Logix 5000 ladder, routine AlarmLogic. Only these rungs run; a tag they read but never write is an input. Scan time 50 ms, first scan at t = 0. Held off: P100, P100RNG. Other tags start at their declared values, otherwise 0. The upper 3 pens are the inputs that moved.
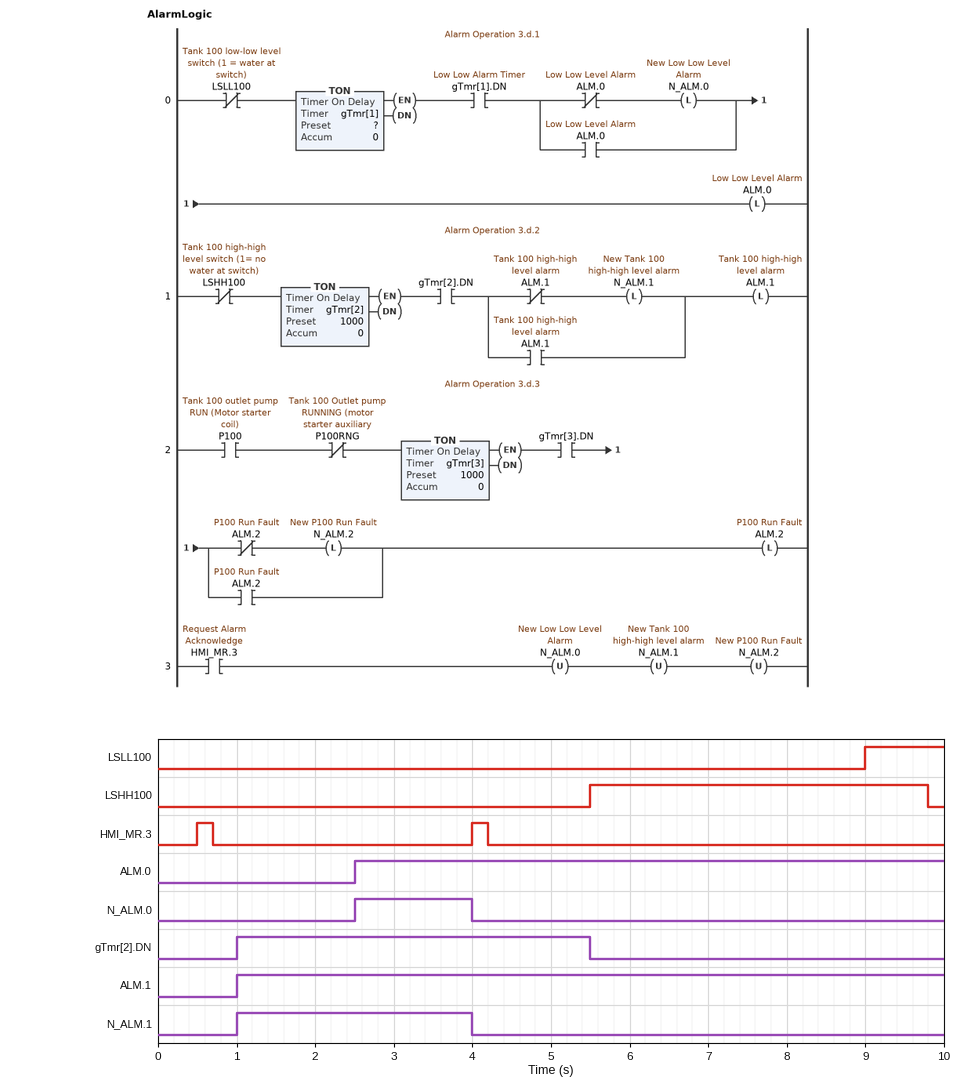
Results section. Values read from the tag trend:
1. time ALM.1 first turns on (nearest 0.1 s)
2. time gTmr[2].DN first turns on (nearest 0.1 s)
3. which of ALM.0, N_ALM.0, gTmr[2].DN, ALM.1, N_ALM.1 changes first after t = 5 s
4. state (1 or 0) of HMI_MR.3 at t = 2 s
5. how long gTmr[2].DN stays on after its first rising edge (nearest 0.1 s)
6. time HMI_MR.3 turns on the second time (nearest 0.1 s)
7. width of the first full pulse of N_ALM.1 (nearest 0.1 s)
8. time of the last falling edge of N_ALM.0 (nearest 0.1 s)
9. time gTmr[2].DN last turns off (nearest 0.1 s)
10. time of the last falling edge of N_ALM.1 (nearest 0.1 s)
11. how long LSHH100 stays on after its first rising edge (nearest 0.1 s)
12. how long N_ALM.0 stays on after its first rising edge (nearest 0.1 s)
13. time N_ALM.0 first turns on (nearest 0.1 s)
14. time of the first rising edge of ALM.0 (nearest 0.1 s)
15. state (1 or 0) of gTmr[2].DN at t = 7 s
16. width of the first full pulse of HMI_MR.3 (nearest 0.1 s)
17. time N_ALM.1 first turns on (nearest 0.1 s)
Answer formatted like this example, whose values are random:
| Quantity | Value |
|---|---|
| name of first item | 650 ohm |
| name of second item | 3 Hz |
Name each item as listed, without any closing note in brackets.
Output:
| Quantity | Value |
|---|---|
| time ALM.1 first turns on | 1.0 s |
| time gTmr[2].DN first turns on | 1.0 s |
| which of ALM.0, N_ALM.0, gTmr[2].DN, ALM.1, N_ALM.1 changes first after t = 5 s | gTmr[2].DN |
| state (1 or 0) of HMI_MR.3 at t = 2 s | 0 |
| how long gTmr[2].DN stays on after its first rising edge | 4.5 s |
| time HMI_MR.3 turns on the second time | 4.0 s |
| width of the first full pulse of N_ALM.1 | 3.0 s |
| time of the last falling edge of N_ALM.0 | 4.0 s |
| time gTmr[2].DN last turns off | 5.5 s |
| time of the last falling edge of N_ALM.1 | 4.0 s |
| how long LSHH100 stays on after its first rising edge | 4.3 s |
| how long N_ALM.0 stays on after its first rising edge | 1.5 s |
| time N_ALM.0 first turns on | 2.5 s |
| time of the first rising edge of ALM.0 | 2.5 s |
| state (1 or 0) of gTmr[2].DN at t = 7 s | 0 |
| width of the first full pulse of HMI_MR.3 | 0.2 s |
| time N_ALM.1 first turns on | 1.0 s |
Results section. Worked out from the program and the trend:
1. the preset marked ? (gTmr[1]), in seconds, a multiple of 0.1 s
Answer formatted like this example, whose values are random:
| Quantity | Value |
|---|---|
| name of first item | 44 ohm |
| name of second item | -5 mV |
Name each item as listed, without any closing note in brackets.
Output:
| Quantity | Value |
|---|---|
| the preset marked ? (gTmr[1]), in seconds, a multiple of 0.1 s | 2.5 s |
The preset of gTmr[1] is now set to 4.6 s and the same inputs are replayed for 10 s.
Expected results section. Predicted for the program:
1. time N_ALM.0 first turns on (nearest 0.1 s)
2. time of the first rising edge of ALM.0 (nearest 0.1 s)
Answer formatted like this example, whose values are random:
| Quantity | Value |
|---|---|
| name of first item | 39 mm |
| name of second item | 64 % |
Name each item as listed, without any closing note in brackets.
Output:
| Quantity | Value |
|---|---|
| time N_ALM.0 first turns on | 4.6 s |
| time of the first rising edge of ALM.0 | 4.6 s |
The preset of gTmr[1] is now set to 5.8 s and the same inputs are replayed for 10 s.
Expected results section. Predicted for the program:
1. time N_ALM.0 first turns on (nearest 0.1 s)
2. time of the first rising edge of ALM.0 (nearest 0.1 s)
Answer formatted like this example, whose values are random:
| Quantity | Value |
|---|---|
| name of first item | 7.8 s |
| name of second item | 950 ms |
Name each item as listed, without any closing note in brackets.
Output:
| Quantity | Value |
|---|---|
| time N_ALM.0 first turns on | 5.8 s |
| time of the first rising edge of ALM.0 | 5.8 s |
